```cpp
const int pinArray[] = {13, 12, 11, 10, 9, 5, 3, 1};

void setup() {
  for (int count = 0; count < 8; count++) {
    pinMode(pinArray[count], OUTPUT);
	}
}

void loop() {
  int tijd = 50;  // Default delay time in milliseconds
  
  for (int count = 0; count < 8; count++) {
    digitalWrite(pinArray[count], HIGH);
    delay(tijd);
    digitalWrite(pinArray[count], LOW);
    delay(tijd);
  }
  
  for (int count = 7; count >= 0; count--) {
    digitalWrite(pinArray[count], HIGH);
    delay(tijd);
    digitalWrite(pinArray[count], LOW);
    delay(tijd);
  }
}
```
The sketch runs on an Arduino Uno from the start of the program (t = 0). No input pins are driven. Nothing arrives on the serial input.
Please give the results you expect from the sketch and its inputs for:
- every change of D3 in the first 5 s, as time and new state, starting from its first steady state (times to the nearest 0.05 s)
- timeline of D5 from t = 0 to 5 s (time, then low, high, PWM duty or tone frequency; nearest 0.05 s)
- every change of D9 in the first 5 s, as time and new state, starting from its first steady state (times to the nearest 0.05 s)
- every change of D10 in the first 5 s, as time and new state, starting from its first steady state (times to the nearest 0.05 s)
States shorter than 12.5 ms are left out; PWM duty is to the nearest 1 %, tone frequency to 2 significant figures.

0 s low; 0.6 s high; 0.65 s low; 0.9 s high; 0.95 s low; 2.2 s high; 2.25 s low; 2.5 s high; 2.55 s low; 3.8 s high; 3.85 s low; 4.1 s high; 4.15 s low
0 s low; 0.5 s high; 0.55 s low; 1 s high; 1.05 s low; 2.1 s high; 2.15 s low; 2.6 s high; 2.65 s low; 3.7 s high; 3.75 s low; 4.2 s high; 4.25 s low
0 s low; 0.4 s high; 0.45 s low; 1.1 s high; 1.15 s low; 2 s high; 2.05 s low; 2.7 s high; 2.75 s low; 3.6 s high; 3.65 s low; 4.3 s high; 4.35 s low
0 s low; 0.3 s high; 0.35 s low; 1.2 s high; 1.25 s low; 1.9 s high; 1.95 s low; 2.8 s high; 2.85 s low; 3.5 s high; 3.55 s low; 4.4 s high; 4.45 s low
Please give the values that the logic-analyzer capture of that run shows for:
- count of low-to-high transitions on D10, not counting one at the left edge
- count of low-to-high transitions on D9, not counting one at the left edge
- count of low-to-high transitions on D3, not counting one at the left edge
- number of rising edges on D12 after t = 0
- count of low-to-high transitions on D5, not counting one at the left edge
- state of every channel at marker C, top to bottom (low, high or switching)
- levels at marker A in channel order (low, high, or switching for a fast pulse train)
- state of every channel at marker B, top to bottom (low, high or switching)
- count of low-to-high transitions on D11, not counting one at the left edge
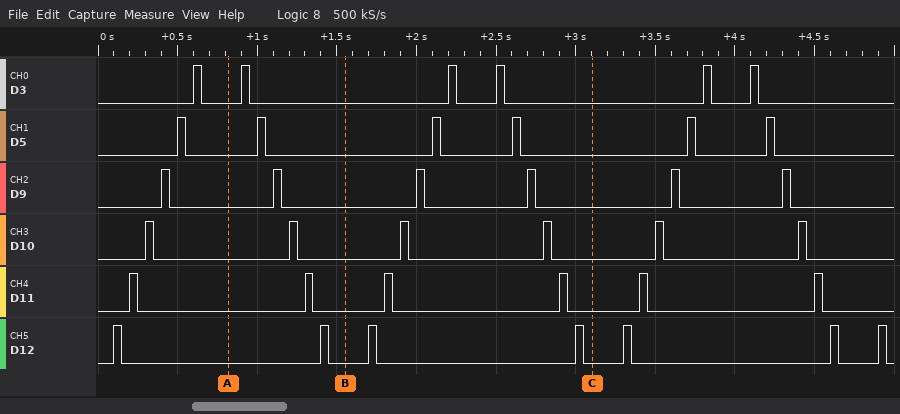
6
6
6
7
6
D3 low, D5 low, D9 low, D10 low, D11 low, D12 low
D3 low, D5 low, D9 low, D10 low, D11 low, D12 low
D3 low, D5 low, D9 low, D10 low, D11 low, D12 low
6
